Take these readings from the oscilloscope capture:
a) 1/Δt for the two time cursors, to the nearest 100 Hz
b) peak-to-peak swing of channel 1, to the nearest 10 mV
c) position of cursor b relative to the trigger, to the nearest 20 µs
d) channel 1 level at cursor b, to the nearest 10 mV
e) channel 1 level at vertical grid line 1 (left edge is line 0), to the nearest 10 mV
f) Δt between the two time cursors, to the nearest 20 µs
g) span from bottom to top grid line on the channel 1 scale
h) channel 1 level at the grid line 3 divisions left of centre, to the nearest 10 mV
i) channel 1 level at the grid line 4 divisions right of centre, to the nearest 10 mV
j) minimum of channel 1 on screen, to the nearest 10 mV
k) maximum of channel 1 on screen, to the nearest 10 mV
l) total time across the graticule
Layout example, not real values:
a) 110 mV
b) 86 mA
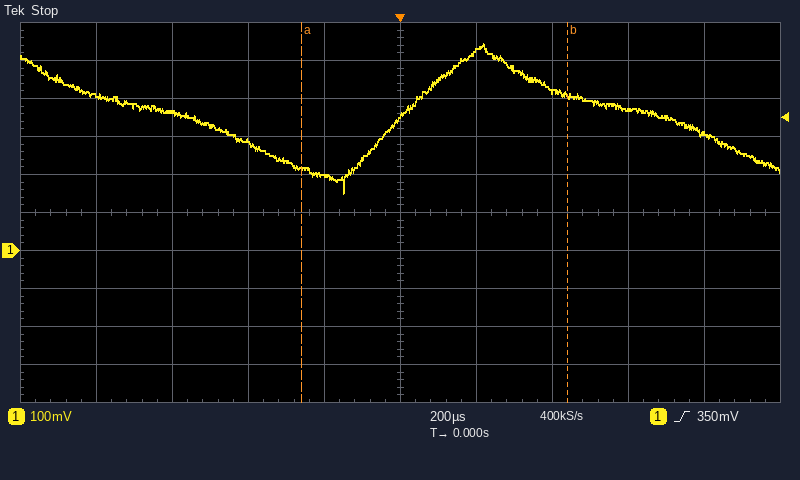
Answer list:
a) 1.4 kHz
b) 390 mV
c) +440 µs
d) 410 mV
e) 410 mV
f) 700 µs
g) 1 V
h) 360 mV
i) 310 mV
j) 150 mV
k) 540 mV
l) 2 ms
